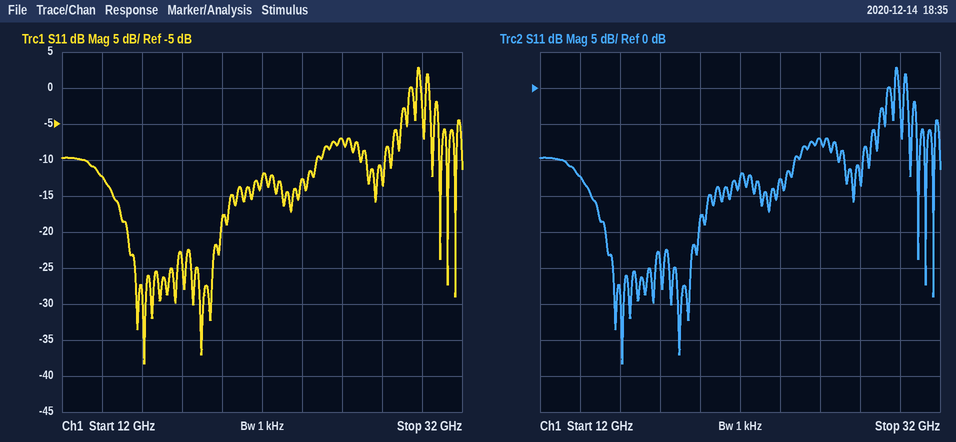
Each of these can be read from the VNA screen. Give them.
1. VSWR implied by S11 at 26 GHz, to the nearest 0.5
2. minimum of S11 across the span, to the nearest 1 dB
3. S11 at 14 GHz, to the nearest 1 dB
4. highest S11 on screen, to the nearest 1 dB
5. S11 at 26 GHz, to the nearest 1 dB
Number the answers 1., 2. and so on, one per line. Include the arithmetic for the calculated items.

1. |Γ| = 10^(-7/20) = 0.4467; VSWR = (1 + 0.4467)/(1 − 0.4467) ≈ 2.61, so 2.5 to the nearest 0.5
2. -38 dB
3. -12 dB
4. 3 dB
5. -7 dB
